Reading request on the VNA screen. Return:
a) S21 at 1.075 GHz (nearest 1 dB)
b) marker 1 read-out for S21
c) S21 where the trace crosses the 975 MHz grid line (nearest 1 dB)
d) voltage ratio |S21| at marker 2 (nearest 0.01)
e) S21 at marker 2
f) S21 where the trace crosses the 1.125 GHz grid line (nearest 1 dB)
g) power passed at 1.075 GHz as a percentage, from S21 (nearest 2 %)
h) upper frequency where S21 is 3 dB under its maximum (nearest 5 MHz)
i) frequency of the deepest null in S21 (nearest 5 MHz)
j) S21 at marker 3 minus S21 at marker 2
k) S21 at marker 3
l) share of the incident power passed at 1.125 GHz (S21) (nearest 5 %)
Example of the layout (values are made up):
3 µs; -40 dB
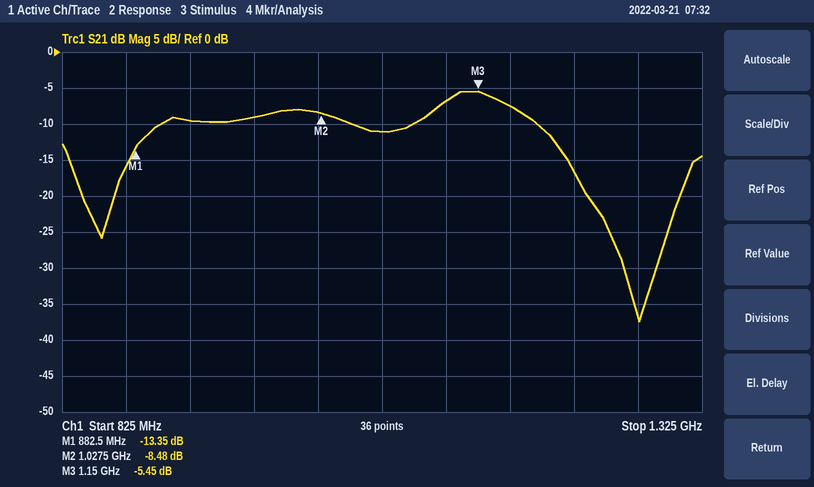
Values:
-11 dB; -13.35 dB; -9 dB; 0.38; -8.48 dB; -7 dB; 8 %; 1.185 GHz; 1.275 GHz; 3.03 dB; -5.45 dB; 20 %
